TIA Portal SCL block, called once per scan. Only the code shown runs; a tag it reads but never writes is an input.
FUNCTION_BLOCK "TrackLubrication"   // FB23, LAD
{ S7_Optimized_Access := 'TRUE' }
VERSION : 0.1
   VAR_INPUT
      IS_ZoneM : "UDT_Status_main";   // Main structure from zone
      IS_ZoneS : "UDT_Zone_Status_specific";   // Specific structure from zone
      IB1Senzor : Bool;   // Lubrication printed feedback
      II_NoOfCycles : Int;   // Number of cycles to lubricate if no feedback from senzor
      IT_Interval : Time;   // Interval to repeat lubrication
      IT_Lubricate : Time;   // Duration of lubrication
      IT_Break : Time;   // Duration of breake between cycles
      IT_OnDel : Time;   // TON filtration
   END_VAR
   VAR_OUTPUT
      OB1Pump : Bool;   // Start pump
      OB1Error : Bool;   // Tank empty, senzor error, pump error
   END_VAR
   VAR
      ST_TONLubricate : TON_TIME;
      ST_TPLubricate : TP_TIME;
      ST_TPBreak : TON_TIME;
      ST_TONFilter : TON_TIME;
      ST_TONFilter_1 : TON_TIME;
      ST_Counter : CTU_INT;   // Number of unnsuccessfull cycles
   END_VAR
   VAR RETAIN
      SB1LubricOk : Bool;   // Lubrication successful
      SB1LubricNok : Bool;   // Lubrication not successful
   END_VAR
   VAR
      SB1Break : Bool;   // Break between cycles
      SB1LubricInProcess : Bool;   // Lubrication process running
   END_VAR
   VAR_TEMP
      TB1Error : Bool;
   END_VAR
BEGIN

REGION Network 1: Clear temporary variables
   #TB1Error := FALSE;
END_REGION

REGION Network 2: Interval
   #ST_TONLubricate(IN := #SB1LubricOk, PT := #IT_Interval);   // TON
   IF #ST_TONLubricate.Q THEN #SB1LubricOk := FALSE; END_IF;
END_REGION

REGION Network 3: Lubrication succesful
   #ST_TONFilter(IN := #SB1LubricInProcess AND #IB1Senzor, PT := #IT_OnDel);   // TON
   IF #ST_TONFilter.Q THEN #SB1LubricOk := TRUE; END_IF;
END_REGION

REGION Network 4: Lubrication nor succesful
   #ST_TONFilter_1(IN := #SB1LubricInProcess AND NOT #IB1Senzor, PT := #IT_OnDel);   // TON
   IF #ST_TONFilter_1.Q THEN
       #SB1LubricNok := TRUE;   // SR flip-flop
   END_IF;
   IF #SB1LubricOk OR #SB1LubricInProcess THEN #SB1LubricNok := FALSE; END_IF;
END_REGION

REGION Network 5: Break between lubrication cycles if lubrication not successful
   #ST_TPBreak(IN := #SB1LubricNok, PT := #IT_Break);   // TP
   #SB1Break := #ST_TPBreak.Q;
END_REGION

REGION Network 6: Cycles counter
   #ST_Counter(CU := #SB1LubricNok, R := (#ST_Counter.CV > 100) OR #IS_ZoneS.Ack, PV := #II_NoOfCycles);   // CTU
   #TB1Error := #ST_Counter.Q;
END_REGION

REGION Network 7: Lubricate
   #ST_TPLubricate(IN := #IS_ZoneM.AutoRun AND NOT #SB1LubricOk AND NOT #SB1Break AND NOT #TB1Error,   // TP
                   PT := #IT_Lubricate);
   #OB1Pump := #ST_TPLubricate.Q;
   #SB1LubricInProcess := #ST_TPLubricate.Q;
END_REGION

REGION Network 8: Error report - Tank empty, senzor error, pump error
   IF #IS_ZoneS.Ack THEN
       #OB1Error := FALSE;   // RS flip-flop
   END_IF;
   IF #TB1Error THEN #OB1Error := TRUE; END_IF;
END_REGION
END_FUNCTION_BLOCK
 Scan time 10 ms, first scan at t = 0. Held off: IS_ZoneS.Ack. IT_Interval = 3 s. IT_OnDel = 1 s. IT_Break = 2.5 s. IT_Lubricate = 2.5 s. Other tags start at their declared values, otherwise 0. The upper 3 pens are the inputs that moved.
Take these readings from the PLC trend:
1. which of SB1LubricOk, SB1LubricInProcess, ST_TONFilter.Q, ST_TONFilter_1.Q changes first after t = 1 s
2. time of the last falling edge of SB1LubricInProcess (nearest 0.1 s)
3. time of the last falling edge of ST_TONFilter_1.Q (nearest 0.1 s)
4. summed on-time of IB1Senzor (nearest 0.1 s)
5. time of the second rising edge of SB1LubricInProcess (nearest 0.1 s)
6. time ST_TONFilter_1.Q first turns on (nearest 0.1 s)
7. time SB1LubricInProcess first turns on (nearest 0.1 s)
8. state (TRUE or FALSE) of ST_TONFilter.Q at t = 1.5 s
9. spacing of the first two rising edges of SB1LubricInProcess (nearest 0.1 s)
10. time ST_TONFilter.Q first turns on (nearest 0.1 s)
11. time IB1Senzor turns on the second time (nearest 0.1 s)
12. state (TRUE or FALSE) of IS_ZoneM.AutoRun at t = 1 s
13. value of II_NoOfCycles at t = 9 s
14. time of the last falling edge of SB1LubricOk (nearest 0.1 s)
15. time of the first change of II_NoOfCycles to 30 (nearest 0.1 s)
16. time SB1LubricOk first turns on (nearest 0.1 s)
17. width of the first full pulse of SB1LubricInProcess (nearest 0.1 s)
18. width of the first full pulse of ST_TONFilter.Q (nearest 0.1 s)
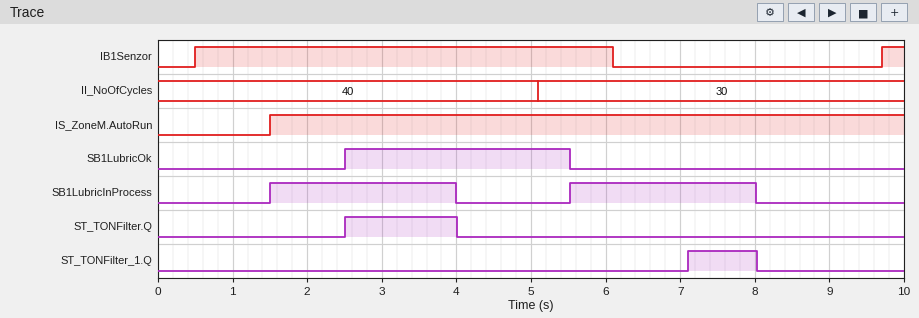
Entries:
SB1LubricInProcess
8.0 s
8.0 s
5.9 s
5.5 s
7.1 s
1.5 s
FALSE
4.0 s
2.5 s
9.7 s
FALSE
30
5.5 s
5.1 s
2.5 s
2.5 s
1.5 s
